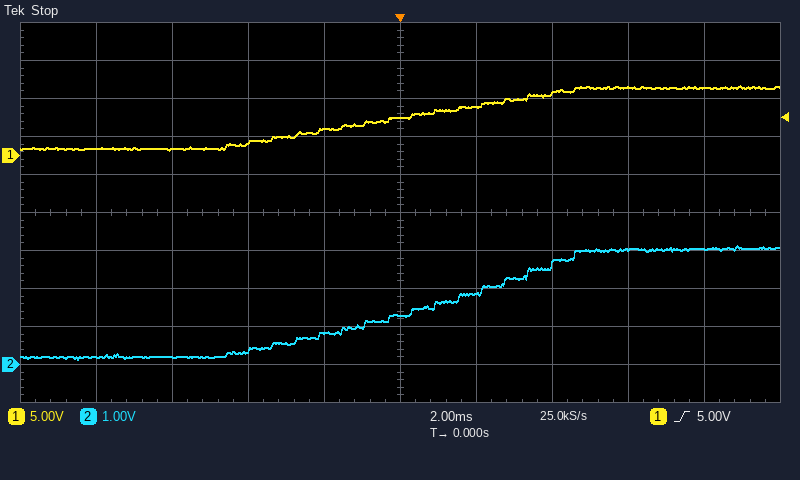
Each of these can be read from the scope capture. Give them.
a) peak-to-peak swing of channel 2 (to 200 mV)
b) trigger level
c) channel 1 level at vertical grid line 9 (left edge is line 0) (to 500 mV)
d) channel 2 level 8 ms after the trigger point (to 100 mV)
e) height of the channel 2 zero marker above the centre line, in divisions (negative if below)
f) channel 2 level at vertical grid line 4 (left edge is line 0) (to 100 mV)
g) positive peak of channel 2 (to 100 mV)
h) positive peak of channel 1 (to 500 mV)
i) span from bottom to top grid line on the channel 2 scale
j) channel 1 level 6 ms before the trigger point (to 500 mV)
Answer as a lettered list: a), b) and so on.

a) 3.0 V
b) 5.00 V
c) 9.0 V
d) 3.0 V
e) -4.0 div
f) 800 mV
g) 3.1 V
h) 9.0 V
i) 10 V
j) 1.0 V
